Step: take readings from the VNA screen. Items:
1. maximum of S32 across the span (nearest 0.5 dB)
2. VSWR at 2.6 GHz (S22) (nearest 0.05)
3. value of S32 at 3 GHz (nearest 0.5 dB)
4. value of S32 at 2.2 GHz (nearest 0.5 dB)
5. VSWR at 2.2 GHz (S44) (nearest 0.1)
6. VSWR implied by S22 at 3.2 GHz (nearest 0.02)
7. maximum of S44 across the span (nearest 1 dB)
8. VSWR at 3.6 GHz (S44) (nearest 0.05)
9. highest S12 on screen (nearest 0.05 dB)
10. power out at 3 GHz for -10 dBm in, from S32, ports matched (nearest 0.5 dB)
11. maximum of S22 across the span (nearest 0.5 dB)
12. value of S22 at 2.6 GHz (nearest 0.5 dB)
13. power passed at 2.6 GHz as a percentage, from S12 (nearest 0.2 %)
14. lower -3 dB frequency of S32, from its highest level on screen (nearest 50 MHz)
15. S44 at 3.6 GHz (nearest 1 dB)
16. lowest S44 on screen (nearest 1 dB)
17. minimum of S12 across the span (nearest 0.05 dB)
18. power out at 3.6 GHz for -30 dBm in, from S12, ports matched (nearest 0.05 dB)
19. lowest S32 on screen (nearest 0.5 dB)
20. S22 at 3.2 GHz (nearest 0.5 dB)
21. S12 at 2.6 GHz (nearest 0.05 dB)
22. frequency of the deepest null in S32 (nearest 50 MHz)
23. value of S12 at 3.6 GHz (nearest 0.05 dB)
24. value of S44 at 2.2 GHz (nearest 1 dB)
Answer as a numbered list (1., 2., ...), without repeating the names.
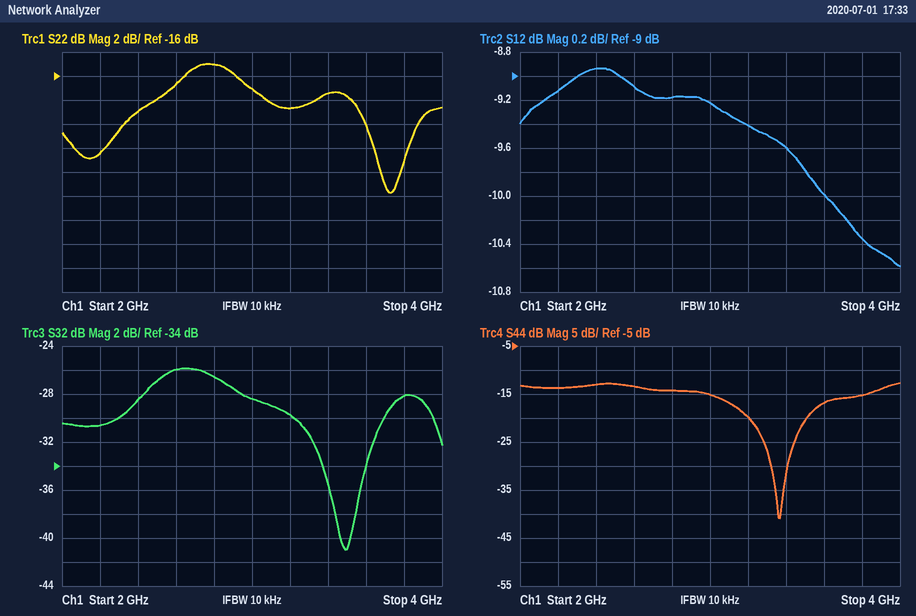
1. -26.0 dB
2. 1.35
3. -28.5 dB
4. -30.5 dB
5. 1.5
6. 1.26
7. -13 dB
8. 1.35
9. -8.95 dB
10. -38.5 dBm
11. -15.0 dB
12. -16.5 dB
13. 12.4 %
14. 2.40 GHz
15. -17 dB
16. -41 dB
17. -10.60 dB
18. -40.00 dBm
19. -41.0 dB
20. -18.5 dB
21. -9.10 dB
22. 3.50 GHz
23. -10.00 dB
24. -14 dB
